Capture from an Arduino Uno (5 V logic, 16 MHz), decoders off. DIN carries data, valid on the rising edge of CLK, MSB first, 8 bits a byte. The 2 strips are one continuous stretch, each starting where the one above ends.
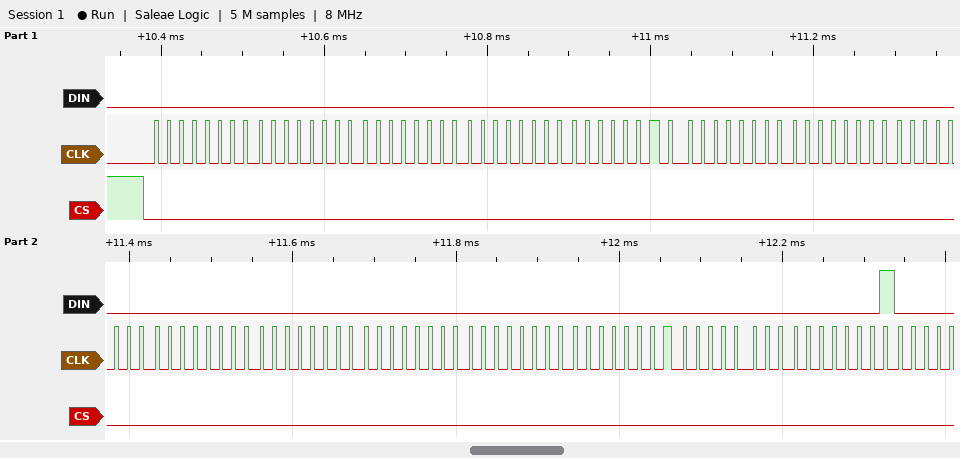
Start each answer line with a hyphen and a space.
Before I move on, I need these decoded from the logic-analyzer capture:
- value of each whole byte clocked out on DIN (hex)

- 00 00 00 00 00 00 00 00 00 00 00 00 00 00 01
